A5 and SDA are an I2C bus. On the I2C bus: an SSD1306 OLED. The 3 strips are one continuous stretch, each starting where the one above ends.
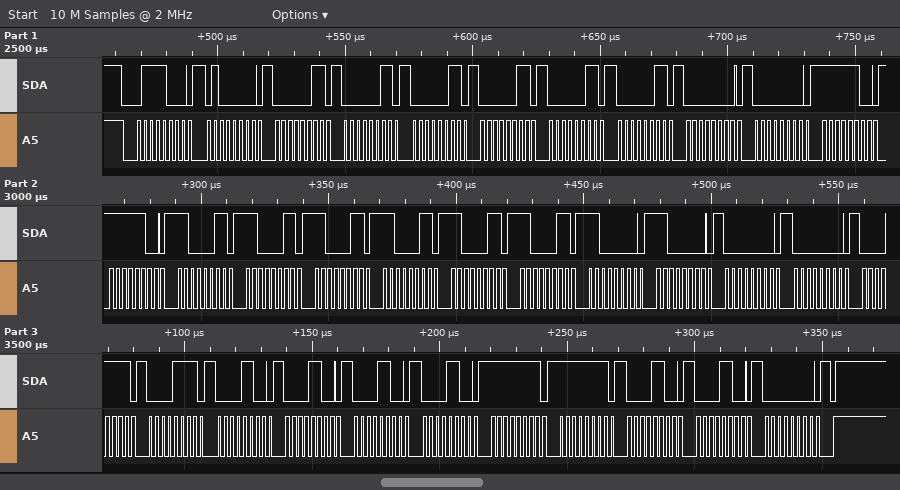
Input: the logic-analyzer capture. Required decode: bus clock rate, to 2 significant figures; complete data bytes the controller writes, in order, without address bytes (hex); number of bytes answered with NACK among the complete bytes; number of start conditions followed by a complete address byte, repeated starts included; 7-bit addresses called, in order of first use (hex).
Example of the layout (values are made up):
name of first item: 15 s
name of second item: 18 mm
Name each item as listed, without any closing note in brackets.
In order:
bus clock rate, to 2 significant figures: 400 kHz
complete data bytes the controller writes, in order, without address bytes: 40 03 03 03 03 03 03 00 00 FC FC C3 C3 C3 C3 C3 C3 C0 C0 00 00 0F 0F 0C 0C 0C 0C FF FF 0C 0C 00
number of bytes answered with NACK among the complete bytes: 0
number of start conditions followed by a complete address byte, repeated starts included: 1
7-bit addresses called, in order of first use: 0x3C
